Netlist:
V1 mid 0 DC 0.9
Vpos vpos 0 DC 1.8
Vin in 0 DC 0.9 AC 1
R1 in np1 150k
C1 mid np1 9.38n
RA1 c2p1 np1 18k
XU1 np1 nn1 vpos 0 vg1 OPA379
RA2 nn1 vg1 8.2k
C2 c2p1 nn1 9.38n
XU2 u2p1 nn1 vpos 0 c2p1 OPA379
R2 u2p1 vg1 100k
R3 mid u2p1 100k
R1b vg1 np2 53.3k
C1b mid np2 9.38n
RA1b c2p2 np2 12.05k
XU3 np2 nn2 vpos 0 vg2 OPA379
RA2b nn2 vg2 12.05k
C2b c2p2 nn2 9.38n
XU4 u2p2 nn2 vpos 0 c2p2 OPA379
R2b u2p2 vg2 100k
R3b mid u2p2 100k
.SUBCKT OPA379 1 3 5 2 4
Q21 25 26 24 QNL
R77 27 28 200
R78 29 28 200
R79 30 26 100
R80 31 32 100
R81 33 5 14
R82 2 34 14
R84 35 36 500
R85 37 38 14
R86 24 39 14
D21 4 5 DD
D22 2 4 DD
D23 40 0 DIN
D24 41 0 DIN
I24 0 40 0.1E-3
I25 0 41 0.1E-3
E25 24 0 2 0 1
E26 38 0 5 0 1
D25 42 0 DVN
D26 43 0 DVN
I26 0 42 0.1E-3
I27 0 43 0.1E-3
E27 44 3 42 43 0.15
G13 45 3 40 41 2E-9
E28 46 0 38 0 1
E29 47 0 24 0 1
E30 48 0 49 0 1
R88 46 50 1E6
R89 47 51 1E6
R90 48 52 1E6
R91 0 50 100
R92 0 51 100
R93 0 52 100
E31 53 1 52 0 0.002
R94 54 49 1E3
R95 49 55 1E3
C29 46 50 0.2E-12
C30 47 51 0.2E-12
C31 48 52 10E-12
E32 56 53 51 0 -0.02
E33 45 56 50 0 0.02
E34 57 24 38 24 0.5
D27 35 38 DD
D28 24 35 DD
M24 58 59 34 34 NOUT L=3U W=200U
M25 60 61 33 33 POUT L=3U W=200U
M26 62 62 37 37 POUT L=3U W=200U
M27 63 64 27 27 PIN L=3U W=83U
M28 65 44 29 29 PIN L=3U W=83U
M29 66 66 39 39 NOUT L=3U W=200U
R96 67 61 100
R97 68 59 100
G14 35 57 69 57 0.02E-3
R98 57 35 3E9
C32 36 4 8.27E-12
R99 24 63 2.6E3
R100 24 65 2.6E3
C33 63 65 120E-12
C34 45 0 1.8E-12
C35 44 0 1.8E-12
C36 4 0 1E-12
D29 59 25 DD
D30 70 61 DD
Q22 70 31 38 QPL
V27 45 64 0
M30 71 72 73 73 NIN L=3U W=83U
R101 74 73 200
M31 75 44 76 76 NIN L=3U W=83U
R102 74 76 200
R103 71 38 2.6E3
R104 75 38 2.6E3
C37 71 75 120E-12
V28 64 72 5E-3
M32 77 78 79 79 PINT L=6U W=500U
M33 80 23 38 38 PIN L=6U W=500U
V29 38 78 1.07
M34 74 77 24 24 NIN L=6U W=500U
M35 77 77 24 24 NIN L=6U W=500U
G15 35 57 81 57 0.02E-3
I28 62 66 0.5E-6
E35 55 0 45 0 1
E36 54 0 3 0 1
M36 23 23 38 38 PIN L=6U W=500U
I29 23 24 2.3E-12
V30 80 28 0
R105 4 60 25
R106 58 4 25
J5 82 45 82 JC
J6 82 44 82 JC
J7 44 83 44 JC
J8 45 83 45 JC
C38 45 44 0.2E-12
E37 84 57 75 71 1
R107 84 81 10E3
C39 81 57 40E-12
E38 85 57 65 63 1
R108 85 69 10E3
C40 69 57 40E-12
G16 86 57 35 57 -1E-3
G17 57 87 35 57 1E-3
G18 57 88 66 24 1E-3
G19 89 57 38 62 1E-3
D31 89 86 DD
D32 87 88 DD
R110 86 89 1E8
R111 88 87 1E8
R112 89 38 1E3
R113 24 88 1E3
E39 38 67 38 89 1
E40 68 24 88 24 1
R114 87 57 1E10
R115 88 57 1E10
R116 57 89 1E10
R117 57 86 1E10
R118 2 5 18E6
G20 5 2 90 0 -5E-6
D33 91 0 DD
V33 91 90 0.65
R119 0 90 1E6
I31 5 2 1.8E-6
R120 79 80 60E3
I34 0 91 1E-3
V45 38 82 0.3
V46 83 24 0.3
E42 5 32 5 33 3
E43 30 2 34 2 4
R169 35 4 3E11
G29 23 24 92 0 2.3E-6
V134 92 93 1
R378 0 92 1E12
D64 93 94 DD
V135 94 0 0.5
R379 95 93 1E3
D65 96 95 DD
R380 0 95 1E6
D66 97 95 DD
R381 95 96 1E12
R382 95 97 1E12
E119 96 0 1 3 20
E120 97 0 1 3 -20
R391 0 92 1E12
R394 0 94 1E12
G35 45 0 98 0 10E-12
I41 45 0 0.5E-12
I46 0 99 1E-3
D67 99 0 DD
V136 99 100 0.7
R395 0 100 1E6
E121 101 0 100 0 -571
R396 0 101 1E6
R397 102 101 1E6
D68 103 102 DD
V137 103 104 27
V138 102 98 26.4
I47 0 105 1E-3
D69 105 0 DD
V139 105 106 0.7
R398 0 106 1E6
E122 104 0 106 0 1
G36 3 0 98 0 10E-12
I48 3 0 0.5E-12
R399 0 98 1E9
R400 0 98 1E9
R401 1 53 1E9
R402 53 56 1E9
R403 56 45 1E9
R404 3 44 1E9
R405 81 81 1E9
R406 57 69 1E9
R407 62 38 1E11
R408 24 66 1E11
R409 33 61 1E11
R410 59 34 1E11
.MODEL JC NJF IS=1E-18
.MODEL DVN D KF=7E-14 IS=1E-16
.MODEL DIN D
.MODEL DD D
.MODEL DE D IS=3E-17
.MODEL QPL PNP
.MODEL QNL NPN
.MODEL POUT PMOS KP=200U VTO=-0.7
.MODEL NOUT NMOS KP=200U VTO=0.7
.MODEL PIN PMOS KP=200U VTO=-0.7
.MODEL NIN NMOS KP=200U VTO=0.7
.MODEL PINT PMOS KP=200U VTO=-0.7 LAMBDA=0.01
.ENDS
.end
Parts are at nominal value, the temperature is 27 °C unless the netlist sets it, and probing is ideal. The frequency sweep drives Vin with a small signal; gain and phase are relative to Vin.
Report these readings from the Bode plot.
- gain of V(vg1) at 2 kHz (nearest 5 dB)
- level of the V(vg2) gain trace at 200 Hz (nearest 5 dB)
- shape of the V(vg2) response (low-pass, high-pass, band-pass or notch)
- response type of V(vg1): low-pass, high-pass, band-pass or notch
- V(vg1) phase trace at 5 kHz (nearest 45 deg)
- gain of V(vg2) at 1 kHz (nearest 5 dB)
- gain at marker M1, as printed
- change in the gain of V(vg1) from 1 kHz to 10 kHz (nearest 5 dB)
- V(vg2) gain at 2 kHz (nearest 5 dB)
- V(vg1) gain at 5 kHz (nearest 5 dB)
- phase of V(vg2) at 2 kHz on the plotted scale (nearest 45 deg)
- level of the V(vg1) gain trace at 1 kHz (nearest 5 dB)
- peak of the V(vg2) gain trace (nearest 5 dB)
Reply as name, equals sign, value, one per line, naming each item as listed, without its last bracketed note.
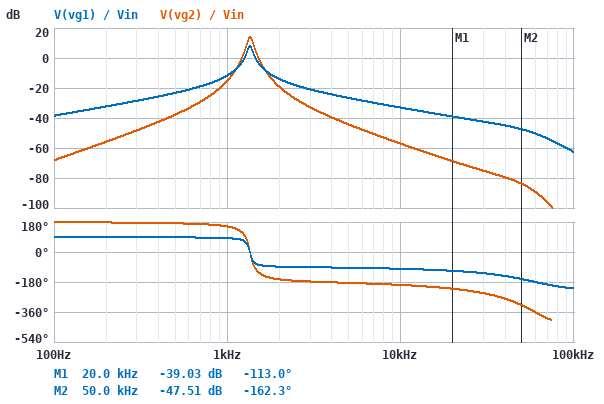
gain of V(vg1) at 2 kHz = -15 dB
level of the V(vg2) gain trace at 200 Hz = -55 dB
shape of the V(vg2) response = band-pass
response type of V(vg1): low-pass, high-pass, band-pass or notch = band-pass
V(vg1) phase trace at 5 kHz = -90 deg
gain of V(vg2) at 1 kHz = -15 dB
gain at marker M1, as printed = -39.03 dB
change in the gain of V(vg1) from 1 kHz to 10 kHz = -20 dB
V(vg2) gain at 2 kHz = -20 dB
V(vg1) gain at 5 kHz = -25 dB
phase of V(vg2) at 2 kHz on the plotted scale = -180 deg
level of the V(vg1) gain trace at 1 kHz = -10 dB
peak of the V(vg2) gain trace = 15 dB
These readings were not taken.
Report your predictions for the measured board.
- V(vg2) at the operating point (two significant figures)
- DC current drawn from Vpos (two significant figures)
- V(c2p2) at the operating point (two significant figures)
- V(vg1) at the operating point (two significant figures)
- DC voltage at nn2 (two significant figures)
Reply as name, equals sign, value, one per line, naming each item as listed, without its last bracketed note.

V(vg2) at the operating point = 890 mV
DC current drawn from Vpos = 9.4 µA
V(c2p2) at the operating point = 900 mV
V(vg1) at the operating point = 890 mV
DC voltage at nn2 = 890 mV
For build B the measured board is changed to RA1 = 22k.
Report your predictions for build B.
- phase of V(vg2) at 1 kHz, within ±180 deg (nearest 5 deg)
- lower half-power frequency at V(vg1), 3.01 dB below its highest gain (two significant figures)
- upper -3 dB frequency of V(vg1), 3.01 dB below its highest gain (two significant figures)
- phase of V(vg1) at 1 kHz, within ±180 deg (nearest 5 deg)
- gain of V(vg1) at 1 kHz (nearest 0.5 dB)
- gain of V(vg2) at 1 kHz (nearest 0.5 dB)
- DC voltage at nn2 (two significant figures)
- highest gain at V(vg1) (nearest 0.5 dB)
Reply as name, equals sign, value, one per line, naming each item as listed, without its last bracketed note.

phase of V(vg2) at 1 kHz, within ±180 deg = 150 deg
lower half-power frequency at V(vg1), 3.01 dB below its highest gain = 1.2 kHz
upper -3 dB frequency of V(vg1), 3.01 dB below its highest gain = 1.3 kHz
phase of V(vg1) at 1 kHz, within ±180 deg = 80 deg
gain of V(vg1) at 1 kHz = -7.5 dB
gain of V(vg2) at 1 kHz = -11.0 dB
DC voltage at nn2 = 890 mV
highest gain at V(vg1) = 7.5 dB
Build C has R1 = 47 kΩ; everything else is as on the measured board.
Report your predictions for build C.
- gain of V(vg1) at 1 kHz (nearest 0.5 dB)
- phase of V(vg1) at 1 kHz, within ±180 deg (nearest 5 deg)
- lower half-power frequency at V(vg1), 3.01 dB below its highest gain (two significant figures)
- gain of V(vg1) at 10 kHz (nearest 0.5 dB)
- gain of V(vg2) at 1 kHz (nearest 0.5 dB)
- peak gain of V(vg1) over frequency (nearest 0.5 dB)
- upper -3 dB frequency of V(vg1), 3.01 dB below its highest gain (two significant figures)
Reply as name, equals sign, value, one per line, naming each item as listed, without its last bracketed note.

gain of V(vg1) at 1 kHz = -2.0 dB
phase of V(vg1) at 1 kHz, within ±180 deg = 65 deg
lower half-power frequency at V(vg1), 3.01 dB below its highest gain = 1.2 kHz
gain of V(vg1) at 10 kHz = -23.0 dB
gain of V(vg2) at 1 kHz = -5.5 dB
peak gain of V(vg1) over frequency = 6.5 dB
upper -3 dB frequency of V(vg1), 3.01 dB below its highest gain = 1.5 kHz
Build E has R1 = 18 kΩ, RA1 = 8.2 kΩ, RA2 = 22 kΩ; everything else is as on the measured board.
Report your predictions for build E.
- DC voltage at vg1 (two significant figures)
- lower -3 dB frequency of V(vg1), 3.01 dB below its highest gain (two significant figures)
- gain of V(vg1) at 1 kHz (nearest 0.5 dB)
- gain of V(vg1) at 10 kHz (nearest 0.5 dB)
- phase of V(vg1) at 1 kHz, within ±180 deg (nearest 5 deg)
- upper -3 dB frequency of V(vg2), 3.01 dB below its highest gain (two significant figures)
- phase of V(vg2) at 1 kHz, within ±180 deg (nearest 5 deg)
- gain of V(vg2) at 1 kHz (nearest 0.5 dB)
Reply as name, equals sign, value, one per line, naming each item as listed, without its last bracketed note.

DC voltage at vg1 = 890 mV
lower -3 dB frequency of V(vg1), 3.01 dB below its highest gain = 850 Hz
gain of V(vg1) at 1 kHz = 5.0 dB
gain of V(vg1) at 10 kHz = -14.5 dB
phase of V(vg1) at 1 kHz, within ±180 deg = 30 deg
upper -3 dB frequency of V(vg2), 3.01 dB below its highest gain = 1.5 kHz
phase of V(vg2) at 1 kHz, within ±180 deg = 100 deg
gain of V(vg2) at 1 kHz = 1.5 dB
